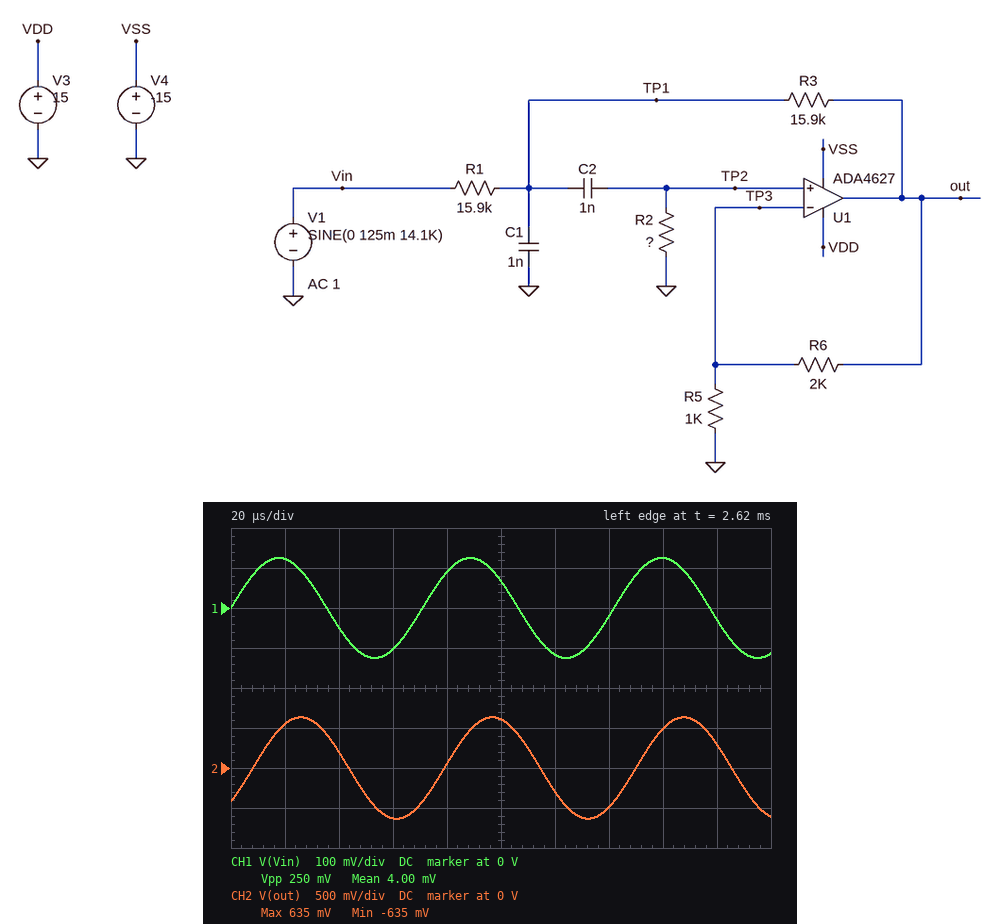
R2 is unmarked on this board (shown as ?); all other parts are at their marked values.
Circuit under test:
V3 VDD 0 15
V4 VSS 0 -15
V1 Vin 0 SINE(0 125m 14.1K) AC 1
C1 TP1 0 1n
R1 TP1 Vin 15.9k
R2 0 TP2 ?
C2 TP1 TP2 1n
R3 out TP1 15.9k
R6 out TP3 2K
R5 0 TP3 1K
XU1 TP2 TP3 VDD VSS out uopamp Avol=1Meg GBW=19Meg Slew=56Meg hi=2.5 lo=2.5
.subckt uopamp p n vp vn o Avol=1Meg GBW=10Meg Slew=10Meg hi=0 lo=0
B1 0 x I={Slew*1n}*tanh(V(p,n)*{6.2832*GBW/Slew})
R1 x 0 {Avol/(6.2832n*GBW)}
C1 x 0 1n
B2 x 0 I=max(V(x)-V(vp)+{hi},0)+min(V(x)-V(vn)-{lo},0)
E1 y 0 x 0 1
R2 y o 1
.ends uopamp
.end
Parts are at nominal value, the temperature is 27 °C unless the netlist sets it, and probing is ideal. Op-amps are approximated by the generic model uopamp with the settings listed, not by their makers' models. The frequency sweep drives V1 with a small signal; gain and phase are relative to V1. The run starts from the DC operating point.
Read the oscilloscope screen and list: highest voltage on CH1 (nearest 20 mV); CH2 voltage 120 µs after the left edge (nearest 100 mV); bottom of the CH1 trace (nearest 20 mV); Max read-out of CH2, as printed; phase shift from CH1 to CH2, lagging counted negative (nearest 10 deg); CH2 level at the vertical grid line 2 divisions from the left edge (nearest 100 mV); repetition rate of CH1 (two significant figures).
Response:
120 mV
-300 mV
-120 mV
635 mV
-40 deg
200 mV
14 kHz
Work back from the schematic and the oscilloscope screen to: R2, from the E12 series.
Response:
22 kΩ
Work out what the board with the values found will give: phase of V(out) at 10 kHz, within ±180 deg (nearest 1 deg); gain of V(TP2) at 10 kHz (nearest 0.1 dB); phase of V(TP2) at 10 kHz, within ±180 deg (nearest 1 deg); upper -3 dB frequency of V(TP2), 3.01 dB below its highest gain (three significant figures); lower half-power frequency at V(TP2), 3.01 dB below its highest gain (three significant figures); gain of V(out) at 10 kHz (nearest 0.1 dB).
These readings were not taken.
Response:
45 deg
4.0 dB
45 deg
14.4 kHz
9.99 kHz
13.6 dB
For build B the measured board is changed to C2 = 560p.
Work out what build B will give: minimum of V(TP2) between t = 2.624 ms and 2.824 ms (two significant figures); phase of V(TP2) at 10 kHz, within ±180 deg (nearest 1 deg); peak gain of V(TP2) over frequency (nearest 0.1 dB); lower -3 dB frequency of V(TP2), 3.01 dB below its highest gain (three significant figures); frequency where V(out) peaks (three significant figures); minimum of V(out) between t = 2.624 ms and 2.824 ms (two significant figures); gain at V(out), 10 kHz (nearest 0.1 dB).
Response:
-110 mV
57 deg
-0.1 dB
11.8 kHz
16.0 kHz
-340 mV
4.1 dB
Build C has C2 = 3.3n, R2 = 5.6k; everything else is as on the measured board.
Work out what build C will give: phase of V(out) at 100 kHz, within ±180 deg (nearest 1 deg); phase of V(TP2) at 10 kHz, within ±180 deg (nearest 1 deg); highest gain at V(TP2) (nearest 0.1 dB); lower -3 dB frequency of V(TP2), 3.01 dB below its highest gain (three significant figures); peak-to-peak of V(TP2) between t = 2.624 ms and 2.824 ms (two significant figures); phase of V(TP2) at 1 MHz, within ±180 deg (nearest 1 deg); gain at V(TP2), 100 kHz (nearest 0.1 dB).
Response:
-76 deg
15 deg
-8.6 dB
5.33 kHz
92 mV
-88 deg
-20.2 dB
